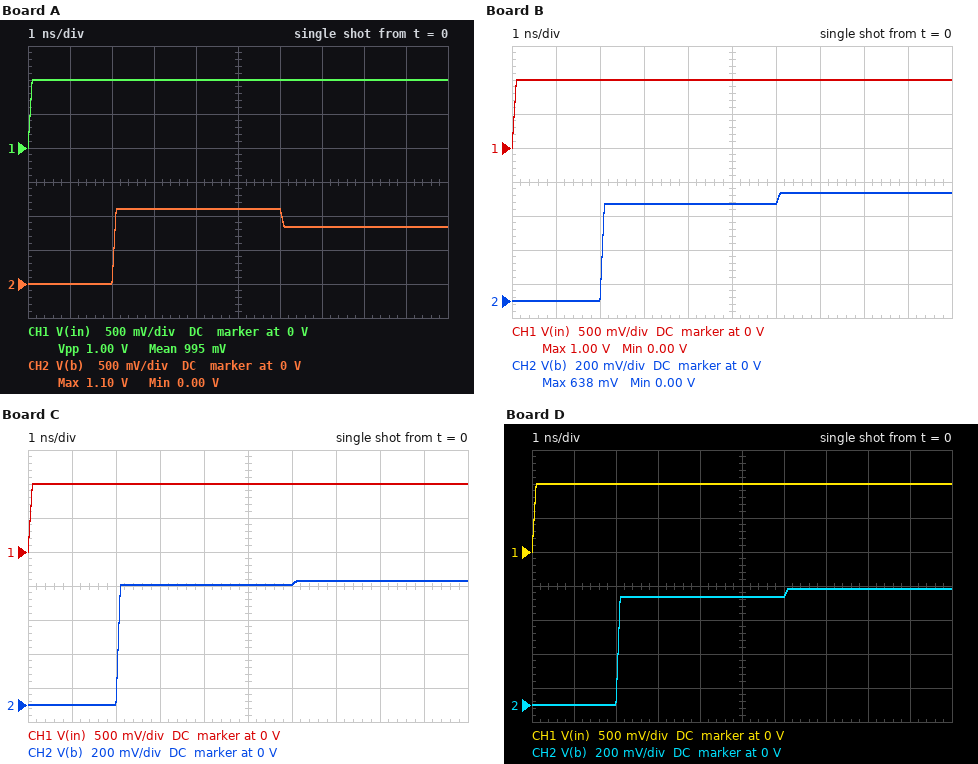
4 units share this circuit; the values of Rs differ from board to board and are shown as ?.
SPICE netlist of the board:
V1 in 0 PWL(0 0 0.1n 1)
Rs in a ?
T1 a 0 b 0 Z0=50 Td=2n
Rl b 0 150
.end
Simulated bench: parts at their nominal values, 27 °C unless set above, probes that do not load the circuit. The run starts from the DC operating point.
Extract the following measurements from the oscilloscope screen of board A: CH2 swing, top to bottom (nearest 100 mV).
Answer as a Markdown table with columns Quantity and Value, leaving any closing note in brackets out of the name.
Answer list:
| Quantity | Value |
|---|---|
| CH2 swing, top to bottom | 1.1 V |
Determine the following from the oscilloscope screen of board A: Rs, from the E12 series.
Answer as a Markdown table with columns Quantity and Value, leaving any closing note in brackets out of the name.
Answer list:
| Quantity | Value |
|---|---|
| Rs, from the E12 series | 18 Ω |
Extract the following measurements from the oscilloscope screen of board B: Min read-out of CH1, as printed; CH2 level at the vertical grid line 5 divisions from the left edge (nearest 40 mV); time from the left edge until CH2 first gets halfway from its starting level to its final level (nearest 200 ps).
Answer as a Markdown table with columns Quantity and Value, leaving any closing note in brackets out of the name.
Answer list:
| Quantity | Value |
|---|---|
| Min read-out of CH1, as printed | 0.00 V |
| CH2 level at the vertical grid line 5 divisions from the left edge | 560 mV |
| time from the left edge until CH2 first gets halfway from its starting level to its final level | 2.0 ns |
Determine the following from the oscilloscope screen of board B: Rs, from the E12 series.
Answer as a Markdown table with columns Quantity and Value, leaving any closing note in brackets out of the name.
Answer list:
| Quantity | Value |
|---|---|
| Rs, from the E12 series | 82 Ω |
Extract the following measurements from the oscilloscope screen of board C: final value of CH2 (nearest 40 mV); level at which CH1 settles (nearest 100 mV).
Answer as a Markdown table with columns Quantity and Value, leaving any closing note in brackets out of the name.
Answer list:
| Quantity | Value |
|---|---|
| final value of CH2 | 720 mV |
| level at which CH1 settles | 1.0 V |
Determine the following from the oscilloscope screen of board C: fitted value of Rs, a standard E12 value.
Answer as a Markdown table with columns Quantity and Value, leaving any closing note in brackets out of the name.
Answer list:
| Quantity | Value |
|---|---|
| fitted value of Rs, a standard E12 value | 56 Ω |
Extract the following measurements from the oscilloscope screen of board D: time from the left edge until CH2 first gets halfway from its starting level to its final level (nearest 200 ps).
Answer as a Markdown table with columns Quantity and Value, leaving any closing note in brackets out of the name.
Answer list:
| Quantity | Value |
|---|---|
| time from the left edge until CH2 first gets halfway from its starting level to its final level | 2.0 ns |
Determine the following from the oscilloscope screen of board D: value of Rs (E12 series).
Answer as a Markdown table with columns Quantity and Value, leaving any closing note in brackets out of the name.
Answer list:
| Quantity | Value |
|---|---|
| value of Rs | 68 Ω |
